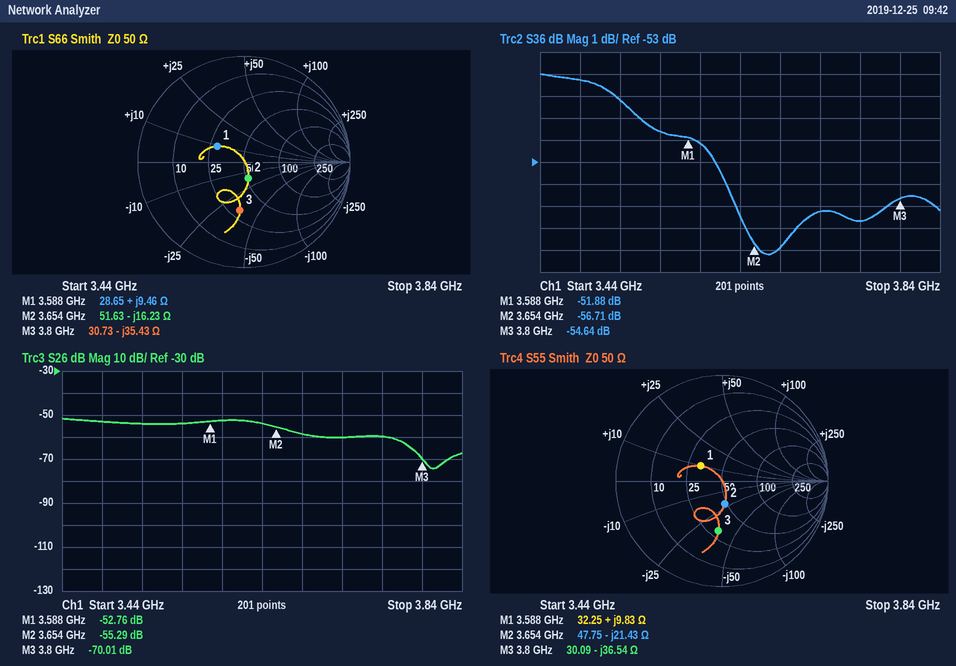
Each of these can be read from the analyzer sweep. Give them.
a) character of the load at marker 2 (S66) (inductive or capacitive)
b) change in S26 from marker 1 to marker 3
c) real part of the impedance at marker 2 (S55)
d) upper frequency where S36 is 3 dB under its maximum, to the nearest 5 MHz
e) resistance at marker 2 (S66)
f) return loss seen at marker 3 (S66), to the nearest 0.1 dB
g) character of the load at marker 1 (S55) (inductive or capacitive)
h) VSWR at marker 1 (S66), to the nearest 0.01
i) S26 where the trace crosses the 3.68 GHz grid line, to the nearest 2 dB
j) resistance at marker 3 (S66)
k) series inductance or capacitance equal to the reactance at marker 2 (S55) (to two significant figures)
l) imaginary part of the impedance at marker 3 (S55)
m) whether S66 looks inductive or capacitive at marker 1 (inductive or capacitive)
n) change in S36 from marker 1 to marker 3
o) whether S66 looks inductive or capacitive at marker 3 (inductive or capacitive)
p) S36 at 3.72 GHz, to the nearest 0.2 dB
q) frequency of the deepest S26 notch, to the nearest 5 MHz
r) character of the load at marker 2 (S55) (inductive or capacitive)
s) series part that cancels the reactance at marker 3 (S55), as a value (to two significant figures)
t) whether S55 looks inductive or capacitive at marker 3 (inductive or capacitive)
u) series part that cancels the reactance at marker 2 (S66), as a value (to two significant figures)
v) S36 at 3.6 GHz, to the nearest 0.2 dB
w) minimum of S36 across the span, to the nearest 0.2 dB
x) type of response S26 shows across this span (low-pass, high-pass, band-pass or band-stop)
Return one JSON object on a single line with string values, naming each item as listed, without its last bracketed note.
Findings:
{"character of the load at marker 2 (S66)": "capacitive", "change in S26 from marker 1 to marker 3": "-17.25 dB", "real part of the impedance at marker 2": "47.75 Ω", "upper frequency where S36 is 3 dB under its maximum, to the nearest 5 MHz": "3.595 GHz", "resistance at marker 2": "51.63 Ω", "return loss seen at marker 3 (S66), to the nearest 0.1 dB": "6.8 dB", "character of the load at marker 1 (S55)": "inductive", "VSWR at marker 1 (S66), to the nearest 0.01": "1.84", "S26 where the trace crosses the 3.68 GHz grid line, to the nearest 2 dB": "-58 dB", "resistance at marker 3": "30.73 Ω", "series inductance or capacitance equal to the reactance at marker 2 (S55)": "2.0 pF", "imaginary part of the impedance at marker 3": "-36.54 Ω", "whether S66 looks inductive or capacitive at marker 1": "inductive", "change in S36 from marker 1 to marker 3": "-2.76 dB", "whether S66 looks inductive or capacitive at marker 3": "capacitive", "S36 at 3.72 GHz, to the nearest 0.2 dB": "-55.2 dB", "frequency of the deepest S26 notch, to the nearest 5 MHz": "3.810 GHz", "character of the load at marker 2 (S55)": "capacitive", "series part that cancels the reactance at marker 3 (S55), as a value": "1.5 nH", "whether S55 looks inductive or capacitive at marker 3": "capacitive", "series part that cancels the reactance at marker 2 (S66), as a value": "710 pH", "S36 at 3.6 GHz, to the nearest 0.2 dB": "-52.2 dB", "minimum of S36 across the span, to the nearest 0.2 dB": "-57.2 dB", "type of response S26 shows across this span": "low-pass"}
